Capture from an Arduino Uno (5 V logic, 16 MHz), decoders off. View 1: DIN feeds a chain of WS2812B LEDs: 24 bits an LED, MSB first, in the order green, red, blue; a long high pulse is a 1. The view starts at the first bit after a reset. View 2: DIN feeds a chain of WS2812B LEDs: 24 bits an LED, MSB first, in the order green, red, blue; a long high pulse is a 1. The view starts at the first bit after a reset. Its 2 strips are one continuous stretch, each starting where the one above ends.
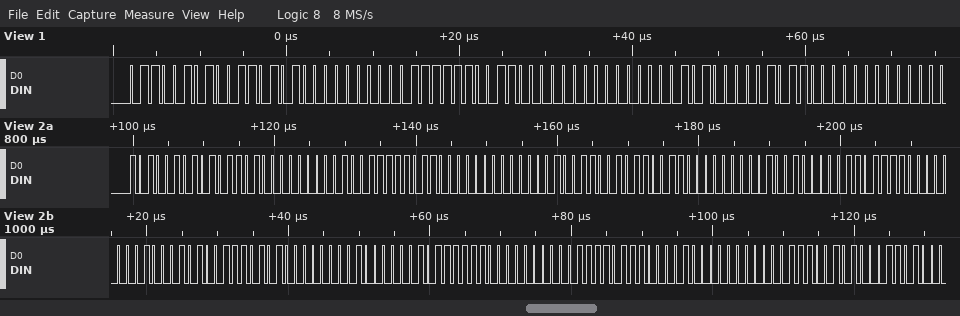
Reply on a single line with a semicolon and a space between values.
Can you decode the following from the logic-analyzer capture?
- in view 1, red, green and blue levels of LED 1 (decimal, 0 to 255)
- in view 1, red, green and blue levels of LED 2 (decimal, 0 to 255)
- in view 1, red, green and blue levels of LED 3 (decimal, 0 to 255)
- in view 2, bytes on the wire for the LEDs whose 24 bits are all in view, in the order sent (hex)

53, 101, 0; 48, 63, 0; 22, 20, 0; A5 5A 00 9F 60 00 99 66 00 90 6F 00 8A 75 00 81 7E 00 7B 84 00
